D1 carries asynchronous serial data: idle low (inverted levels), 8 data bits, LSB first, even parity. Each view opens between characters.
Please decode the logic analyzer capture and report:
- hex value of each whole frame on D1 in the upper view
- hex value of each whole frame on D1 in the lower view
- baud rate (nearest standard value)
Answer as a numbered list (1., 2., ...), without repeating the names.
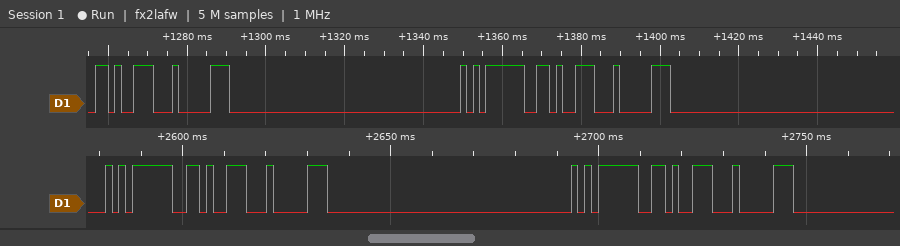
1. 1A, 1F, 05, 1A, 1F
2. 05, 1A, 1F, 05, 1A, 1F
3. 600 baud
